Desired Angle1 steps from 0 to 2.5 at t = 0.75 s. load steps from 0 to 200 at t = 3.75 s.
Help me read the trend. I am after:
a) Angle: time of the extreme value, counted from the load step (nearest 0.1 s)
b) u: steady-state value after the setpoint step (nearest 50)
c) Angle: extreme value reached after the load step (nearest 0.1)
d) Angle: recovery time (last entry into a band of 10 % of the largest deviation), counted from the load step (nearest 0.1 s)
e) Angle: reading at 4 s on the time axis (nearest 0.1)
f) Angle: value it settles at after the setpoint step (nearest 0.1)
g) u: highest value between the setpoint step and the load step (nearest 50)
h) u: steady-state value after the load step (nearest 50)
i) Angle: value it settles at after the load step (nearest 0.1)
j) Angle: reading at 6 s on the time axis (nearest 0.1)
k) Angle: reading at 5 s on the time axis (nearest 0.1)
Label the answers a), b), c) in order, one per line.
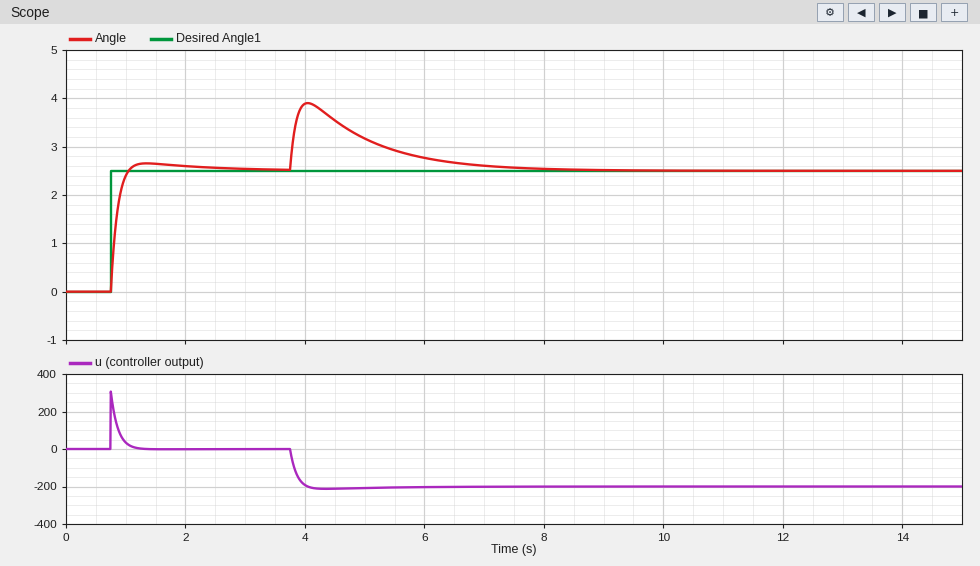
a) 0.3 s
b) 0
c) 3.9
d) 3.0 s
e) 3.9
f) 2.5
g) 300
h) -200
i) 2.5
j) 2.8
k) 3.2
